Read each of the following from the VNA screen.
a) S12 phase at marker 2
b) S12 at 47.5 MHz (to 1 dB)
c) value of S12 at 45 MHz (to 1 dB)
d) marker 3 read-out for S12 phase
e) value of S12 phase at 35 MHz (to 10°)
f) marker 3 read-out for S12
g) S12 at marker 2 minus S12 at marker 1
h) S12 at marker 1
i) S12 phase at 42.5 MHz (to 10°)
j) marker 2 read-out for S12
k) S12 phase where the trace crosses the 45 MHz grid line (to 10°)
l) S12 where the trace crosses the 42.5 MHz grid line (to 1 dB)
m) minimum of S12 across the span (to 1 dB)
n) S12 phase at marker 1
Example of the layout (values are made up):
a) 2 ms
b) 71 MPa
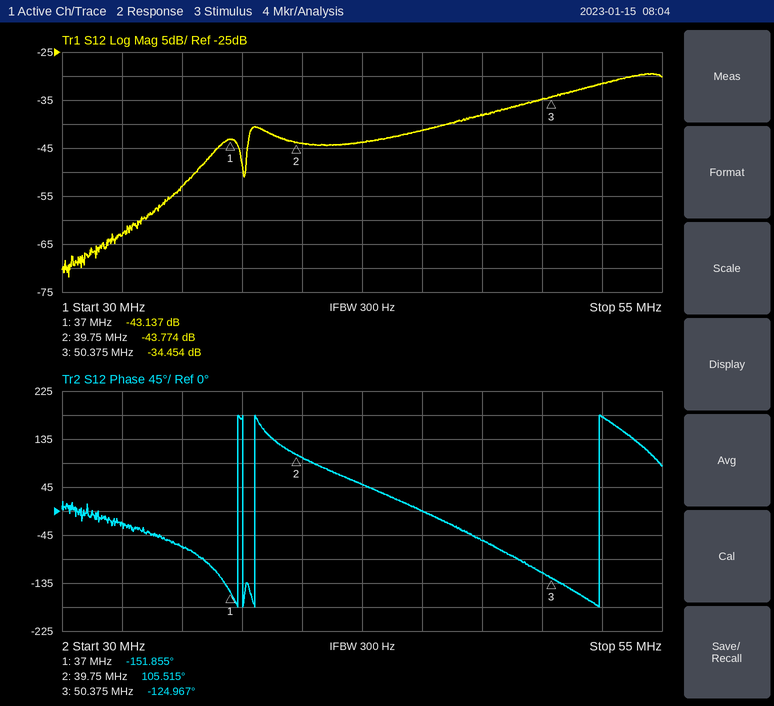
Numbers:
a) 105.515°
b) -38 dB
c) -41 dB
d) -124.967°
e) -70°
f) -34.454 dB
g) -0.637 dB
h) -43.137 dB
i) 50°
j) -43.774 dB
k) 0°
l) -44 dB
m) -72 dB
n) -151.855°
